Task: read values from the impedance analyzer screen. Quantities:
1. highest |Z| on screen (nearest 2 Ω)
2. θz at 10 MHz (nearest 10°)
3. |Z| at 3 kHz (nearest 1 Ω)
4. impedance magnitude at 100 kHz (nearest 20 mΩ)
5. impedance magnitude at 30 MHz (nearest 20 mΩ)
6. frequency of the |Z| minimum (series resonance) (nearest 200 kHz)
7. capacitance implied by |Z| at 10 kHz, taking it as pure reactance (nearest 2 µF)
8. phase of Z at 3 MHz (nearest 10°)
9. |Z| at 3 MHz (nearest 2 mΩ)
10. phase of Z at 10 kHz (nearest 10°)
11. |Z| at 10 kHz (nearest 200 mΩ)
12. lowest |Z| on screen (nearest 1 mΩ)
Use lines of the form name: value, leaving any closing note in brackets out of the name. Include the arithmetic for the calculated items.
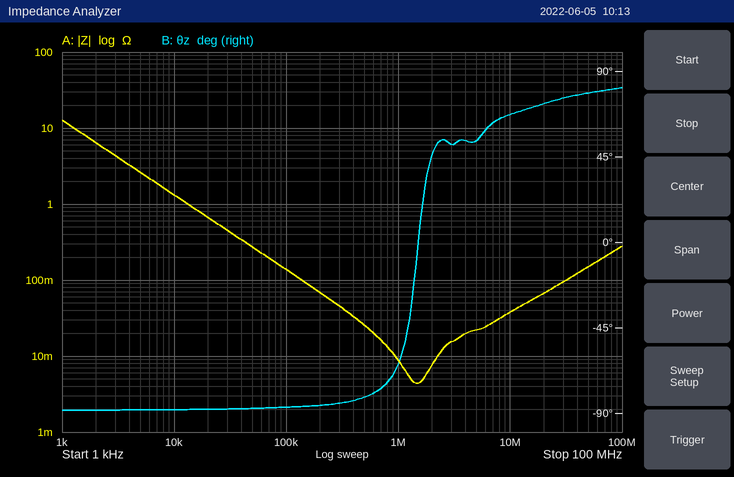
highest |Z| on screen: 12 Ω
θz at 10 MHz: 70°
|Z| at 3 kHz: 4 Ω
impedance magnitude at 100 kHz: 140 mΩ
impedance magnitude at 30 MHz: 100 mΩ
frequency of the |Z| minimum (series resonance): 1.4 MHz
capacitance implied by |Z| at 10 kHz, taking it as pure reactance: C = 1/(2π × 10 kHz × 1.4 Ω) ≈ 11.4 µF, so 12 µF to the nearest 2 µF
phase of Z at 3 MHz: 50°
|Z| at 3 MHz: 16 mΩ
phase of Z at 10 kHz: -90°
|Z| at 10 kHz: 1.4 Ω
lowest |Z| on screen: 4 mΩ
